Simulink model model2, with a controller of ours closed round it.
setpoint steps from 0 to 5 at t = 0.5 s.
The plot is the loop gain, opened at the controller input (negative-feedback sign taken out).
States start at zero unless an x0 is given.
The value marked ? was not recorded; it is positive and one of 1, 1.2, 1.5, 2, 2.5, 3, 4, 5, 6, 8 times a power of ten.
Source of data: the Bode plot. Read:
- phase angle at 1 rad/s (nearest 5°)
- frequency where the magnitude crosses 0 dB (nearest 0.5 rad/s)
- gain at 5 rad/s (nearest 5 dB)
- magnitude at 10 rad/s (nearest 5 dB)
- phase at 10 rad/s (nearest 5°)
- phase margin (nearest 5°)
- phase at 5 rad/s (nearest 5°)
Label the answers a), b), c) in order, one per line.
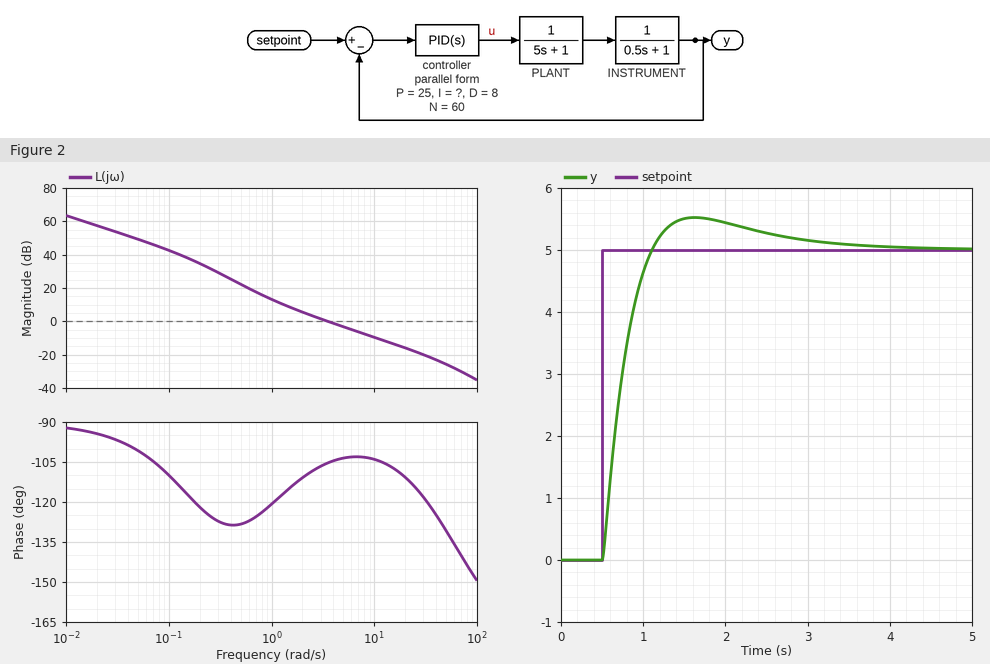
a) -120°
b) 3.5 rad/s
c) -5 dB
d) -10 dB
e) -105°
f) 75°
g) -105°
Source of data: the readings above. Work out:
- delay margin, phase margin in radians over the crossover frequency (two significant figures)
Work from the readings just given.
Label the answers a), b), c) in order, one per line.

a) 0.37 s
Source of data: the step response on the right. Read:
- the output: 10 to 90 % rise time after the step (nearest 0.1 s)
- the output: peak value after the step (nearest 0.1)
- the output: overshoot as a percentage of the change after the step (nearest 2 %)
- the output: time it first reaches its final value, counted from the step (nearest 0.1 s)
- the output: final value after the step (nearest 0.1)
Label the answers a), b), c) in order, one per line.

a) 0.4 s
b) 5.5
c) 10 %
d) 0.6 s
e) 5.0
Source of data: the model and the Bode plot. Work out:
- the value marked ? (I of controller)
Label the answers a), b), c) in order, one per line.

a) 15
